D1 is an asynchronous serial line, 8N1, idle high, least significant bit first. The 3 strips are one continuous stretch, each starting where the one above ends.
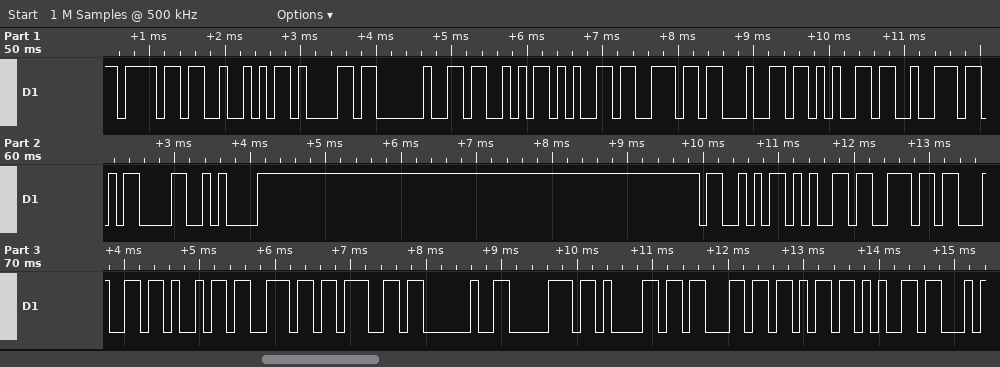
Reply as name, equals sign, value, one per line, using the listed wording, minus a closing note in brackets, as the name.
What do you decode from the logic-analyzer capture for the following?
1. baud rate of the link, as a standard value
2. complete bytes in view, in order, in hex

baud rate of the link, as a standard value = 9600 baud
complete bytes in view, in order, in hex = 6F 52 61 20 53 65 6E 64 65 72 0D 0A 53 65 6E 64 69 6E 67 20 70 61 63 6B 65
